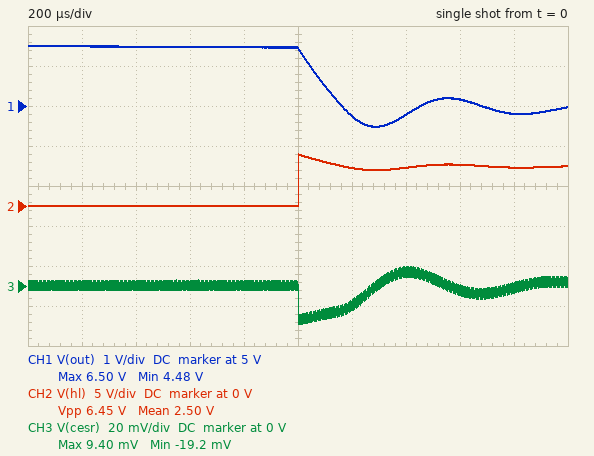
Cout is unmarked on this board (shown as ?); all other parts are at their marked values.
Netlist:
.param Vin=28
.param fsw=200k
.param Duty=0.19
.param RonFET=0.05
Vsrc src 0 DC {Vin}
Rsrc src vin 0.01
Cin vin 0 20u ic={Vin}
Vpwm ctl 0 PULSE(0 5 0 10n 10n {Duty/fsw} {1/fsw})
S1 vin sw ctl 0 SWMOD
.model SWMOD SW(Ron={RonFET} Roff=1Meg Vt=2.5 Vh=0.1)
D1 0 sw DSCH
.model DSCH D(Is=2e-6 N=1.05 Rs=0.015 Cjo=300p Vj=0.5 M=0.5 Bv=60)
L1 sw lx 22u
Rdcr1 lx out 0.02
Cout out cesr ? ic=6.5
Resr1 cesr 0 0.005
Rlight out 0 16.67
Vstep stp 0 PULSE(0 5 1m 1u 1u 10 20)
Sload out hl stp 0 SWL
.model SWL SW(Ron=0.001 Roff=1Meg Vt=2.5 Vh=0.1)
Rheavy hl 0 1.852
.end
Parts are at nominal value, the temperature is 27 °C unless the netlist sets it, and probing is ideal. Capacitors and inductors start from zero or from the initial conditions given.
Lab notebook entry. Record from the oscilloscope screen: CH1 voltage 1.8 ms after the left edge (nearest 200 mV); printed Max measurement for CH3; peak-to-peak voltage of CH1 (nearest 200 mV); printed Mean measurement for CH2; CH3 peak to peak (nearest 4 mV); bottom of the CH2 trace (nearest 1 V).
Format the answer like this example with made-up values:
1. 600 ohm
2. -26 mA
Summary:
1. 4.8 V
2. 9.40 mV
3. 2.0 V
4. 2.50 V
5. 28 mV
6. 0 V
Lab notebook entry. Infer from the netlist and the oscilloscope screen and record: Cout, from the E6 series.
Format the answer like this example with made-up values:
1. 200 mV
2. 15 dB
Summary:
1. 330 µF
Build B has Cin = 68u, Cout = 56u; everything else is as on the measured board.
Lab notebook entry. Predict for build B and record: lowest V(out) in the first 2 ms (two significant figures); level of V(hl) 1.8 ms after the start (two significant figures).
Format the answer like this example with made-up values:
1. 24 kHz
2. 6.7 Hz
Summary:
1. 3.8 V
2. 4.9 V
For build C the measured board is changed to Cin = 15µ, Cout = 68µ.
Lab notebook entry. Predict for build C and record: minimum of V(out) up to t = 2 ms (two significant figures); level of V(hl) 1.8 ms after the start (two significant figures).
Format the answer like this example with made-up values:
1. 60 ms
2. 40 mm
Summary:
1. 3.9 V
2. 4.9 V
